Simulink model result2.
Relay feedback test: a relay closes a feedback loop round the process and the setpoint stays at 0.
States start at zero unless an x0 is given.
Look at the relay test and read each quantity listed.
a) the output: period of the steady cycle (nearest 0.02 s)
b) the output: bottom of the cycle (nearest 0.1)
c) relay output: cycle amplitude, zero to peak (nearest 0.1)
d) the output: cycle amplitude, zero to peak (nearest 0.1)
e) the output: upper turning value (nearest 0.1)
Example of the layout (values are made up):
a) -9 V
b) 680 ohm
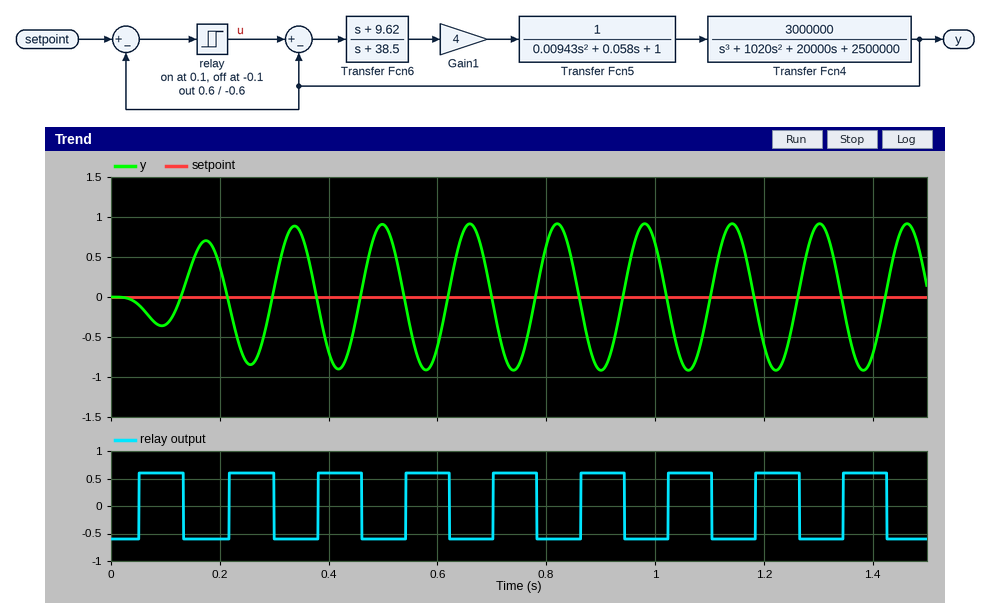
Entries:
a) 0.16 s
b) -0.9
c) 0.6
d) 0.9
e) 0.9
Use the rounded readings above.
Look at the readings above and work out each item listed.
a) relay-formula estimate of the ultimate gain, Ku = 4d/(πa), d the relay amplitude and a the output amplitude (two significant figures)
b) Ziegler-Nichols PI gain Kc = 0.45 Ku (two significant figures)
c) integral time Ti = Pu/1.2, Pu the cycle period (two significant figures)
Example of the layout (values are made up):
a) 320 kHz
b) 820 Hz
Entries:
a) 0.85
b) 0.38
c) 0.13 s
